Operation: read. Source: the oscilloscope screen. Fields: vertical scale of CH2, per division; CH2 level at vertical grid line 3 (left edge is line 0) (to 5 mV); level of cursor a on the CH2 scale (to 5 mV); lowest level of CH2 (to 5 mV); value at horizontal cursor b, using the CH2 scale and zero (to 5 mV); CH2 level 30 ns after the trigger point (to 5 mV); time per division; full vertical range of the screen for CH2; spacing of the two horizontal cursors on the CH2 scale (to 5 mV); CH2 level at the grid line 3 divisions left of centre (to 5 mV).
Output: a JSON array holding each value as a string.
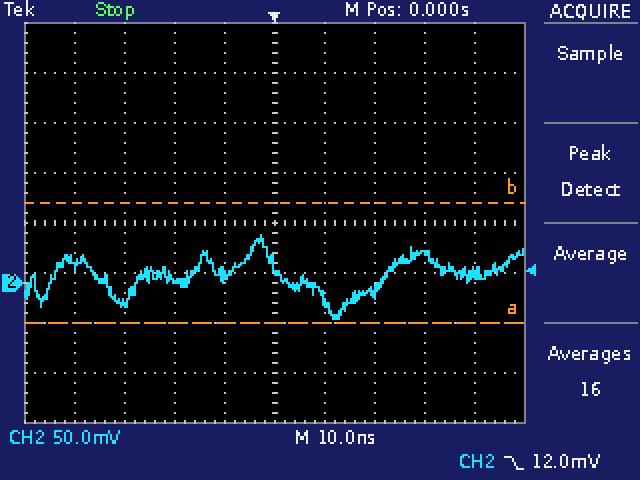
["50 mV", "5 mV", "-40 mV", "-35 mV", "80 mV", "30 mV", "10 ns", "400 mV", "120 mV", "-20 mV"]
